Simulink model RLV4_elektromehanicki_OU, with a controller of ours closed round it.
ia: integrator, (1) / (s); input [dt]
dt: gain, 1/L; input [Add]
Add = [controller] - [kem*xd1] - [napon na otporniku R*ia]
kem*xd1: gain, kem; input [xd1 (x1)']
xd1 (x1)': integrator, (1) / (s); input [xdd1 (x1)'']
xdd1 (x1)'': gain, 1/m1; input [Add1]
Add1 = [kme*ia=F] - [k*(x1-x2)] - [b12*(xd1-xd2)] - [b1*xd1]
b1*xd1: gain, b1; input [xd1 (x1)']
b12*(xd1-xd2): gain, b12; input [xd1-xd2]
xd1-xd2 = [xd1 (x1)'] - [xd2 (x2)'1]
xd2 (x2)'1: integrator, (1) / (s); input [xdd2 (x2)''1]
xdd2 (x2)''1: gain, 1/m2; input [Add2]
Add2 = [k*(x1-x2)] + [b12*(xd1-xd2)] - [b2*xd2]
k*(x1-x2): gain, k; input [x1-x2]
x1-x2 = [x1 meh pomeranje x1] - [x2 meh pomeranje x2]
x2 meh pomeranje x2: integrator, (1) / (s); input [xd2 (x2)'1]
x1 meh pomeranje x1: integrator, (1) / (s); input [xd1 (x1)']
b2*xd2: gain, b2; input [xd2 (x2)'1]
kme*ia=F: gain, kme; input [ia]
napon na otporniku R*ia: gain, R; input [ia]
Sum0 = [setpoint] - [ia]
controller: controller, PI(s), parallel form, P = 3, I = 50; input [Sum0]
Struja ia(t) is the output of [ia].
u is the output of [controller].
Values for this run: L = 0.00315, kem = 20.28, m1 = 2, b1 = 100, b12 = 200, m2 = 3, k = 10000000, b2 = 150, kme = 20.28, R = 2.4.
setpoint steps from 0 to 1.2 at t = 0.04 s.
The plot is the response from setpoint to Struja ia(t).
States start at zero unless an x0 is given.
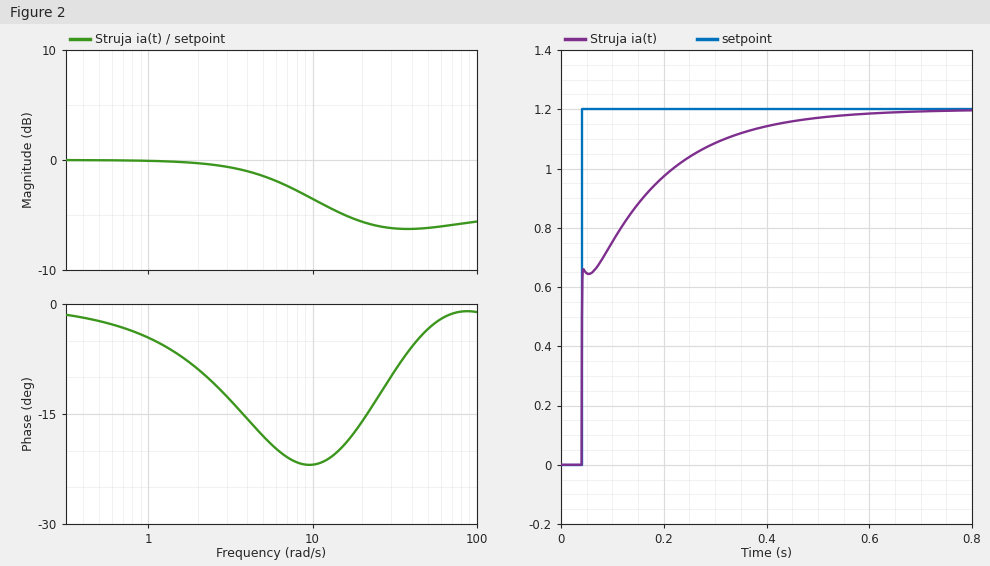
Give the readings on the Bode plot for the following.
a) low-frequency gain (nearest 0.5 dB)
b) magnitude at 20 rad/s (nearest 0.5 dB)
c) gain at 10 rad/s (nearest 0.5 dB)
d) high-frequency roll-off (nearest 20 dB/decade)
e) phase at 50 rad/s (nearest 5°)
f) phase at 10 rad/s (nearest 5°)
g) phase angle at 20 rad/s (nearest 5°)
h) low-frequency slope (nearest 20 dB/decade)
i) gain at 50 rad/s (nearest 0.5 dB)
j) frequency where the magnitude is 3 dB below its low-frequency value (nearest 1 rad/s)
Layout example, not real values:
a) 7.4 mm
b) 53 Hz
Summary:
a) 0.0 dB
b) -5.5 dB
c) -3.5 dB
d) 0 dB/decade
e) -5°
f) -20°
g) -15°
h) 0 dB/decade
i) -6.0 dB
j) 9 rad/s
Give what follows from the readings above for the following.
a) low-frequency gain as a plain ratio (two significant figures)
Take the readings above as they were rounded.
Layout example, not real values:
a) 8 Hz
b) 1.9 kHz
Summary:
a) 1.0
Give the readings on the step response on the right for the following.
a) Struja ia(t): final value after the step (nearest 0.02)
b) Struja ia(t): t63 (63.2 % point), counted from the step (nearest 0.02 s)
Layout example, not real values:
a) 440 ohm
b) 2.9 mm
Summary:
a) 1.20
b) 0.06 s
